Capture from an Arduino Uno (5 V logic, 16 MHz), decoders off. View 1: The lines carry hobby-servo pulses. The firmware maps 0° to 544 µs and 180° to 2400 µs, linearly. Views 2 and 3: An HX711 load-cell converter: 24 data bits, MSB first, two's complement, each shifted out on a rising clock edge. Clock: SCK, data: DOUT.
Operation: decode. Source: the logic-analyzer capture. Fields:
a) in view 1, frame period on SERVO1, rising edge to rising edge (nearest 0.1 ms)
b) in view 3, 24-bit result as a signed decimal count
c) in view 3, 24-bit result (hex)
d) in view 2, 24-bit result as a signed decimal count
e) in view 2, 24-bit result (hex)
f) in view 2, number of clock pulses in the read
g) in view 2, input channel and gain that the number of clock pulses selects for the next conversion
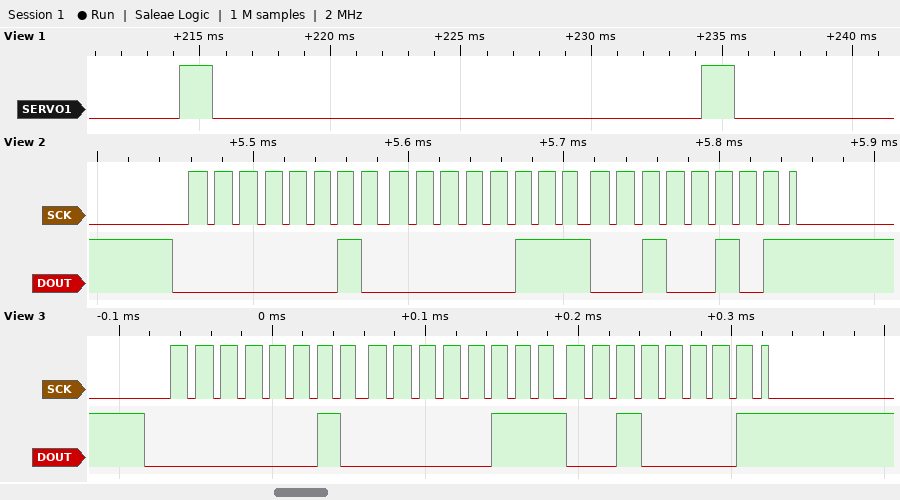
20.0 ms
132897
0x020721
132901
0x020725
25
channel A, gain 128
